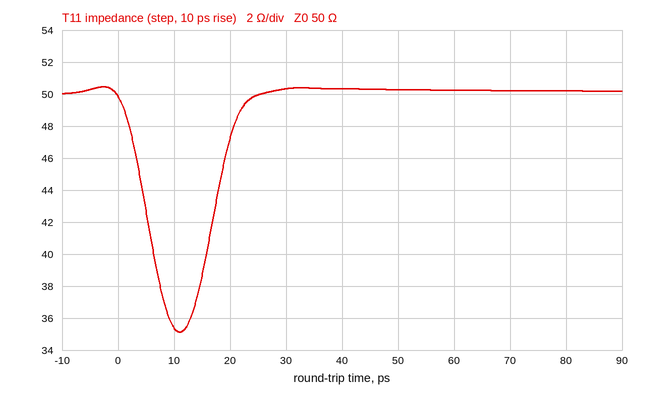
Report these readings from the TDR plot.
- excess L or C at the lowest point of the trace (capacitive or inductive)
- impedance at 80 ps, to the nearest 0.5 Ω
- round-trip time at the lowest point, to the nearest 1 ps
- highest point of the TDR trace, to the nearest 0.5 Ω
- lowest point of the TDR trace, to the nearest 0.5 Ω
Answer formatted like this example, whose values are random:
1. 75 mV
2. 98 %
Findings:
1. capacitive
2. 50.0 Ω
3. 11 ps
4. 50.5 Ω
5. 35.0 Ω
